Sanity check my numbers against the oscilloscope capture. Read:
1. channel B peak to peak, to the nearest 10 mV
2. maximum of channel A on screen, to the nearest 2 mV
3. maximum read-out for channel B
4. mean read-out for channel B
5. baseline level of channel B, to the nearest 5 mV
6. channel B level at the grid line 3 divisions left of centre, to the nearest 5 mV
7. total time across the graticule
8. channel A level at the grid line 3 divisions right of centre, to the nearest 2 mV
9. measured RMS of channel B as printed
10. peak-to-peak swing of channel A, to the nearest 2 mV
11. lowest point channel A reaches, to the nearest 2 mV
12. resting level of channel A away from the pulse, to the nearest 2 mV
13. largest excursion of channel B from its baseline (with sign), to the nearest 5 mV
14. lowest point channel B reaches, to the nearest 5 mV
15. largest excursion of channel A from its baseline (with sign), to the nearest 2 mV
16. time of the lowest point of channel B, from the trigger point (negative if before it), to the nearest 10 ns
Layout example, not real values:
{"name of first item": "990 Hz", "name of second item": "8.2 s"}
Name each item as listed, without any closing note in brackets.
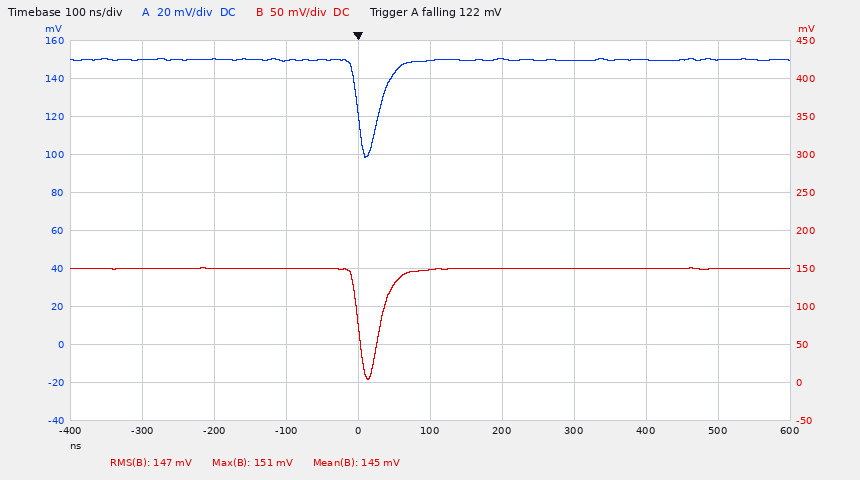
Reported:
{"channel B peak to peak, to the nearest 10 mV": "150 mV", "maximum of channel A on screen, to the nearest 2 mV": "150 mV", "maximum read-out for channel B": "151 mV", "mean read-out for channel B": "145 mV", "baseline level of channel B, to the nearest 5 mV": "150 mV", "channel B level at the grid line 3 divisions left of centre, to the nearest 5 mV": "150 mV", "total time across the graticule": "1 µs", "channel A level at the grid line 3 divisions right of centre, to the nearest 2 mV": "150 mV", "measured RMS of channel B as printed": "147 mV", "peak-to-peak swing of channel A, to the nearest 2 mV": "52 mV", "lowest point channel A reaches, to the nearest 2 mV": "98 mV", "resting level of channel A away from the pulse, to the nearest 2 mV": "150 mV", "largest excursion of channel B from its baseline (with sign), to the nearest 5 mV": "-145 mV", "lowest point channel B reaches, to the nearest 5 mV": "5 mV", "largest excursion of channel A from its baseline (with sign), to the nearest 2 mV": "-52 mV", "time of the lowest point of channel B, from the trigger point (negative if before it), to the nearest 10 ns": "+10 ns"}
